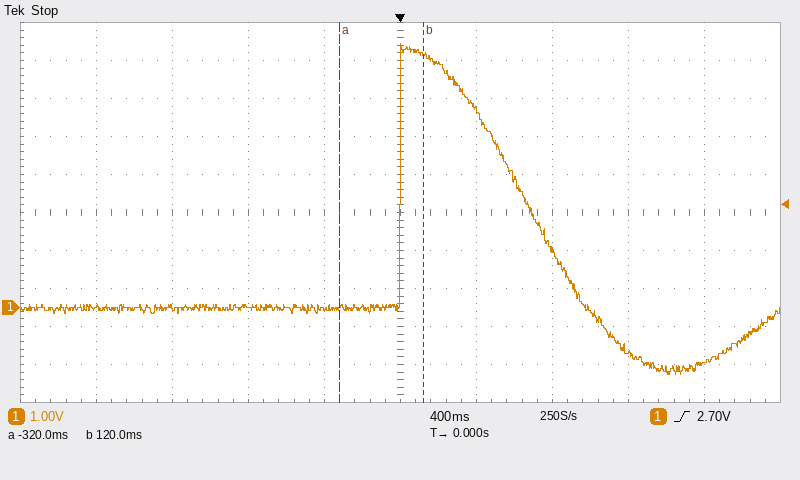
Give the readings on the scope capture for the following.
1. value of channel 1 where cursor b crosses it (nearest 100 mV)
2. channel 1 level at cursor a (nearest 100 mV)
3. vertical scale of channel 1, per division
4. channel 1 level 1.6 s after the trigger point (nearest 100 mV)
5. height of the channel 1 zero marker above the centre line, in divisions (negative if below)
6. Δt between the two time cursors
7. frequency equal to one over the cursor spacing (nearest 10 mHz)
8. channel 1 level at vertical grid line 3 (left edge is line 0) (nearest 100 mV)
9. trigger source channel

6.6 V
0.0 V
1 V
-1.4 V
-2.5 div
440 ms
2.27 Hz
0.0 V
channel 1
